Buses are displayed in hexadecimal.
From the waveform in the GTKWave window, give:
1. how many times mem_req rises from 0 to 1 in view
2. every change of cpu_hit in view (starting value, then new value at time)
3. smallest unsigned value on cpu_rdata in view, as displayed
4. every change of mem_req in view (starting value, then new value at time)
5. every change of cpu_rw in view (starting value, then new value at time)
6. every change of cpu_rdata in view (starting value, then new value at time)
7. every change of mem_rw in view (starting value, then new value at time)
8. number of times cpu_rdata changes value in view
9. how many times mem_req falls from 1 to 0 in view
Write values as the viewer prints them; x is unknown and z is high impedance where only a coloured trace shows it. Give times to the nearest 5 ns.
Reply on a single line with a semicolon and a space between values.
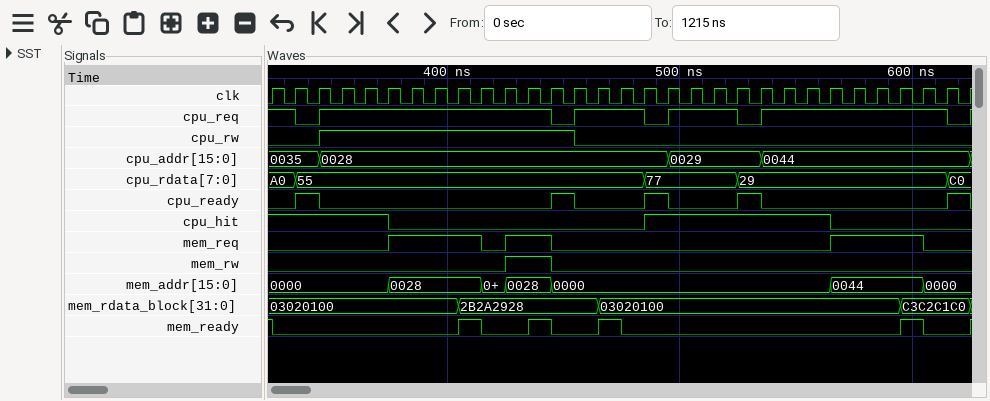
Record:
3; 1, 0 at 375 ns, 1 at 485 ns, 0 at 565 ns; 29; 0, 1 at 375 ns, 0 at 415 ns, 1 at 425 ns, 0 at 445 ns, 1 at 565 ns, 0 at 605 ns; 0, 1 at 345 ns, 0 at 455 ns; A0, 55 at 335 ns, 77 at 485 ns, 29 at 525 ns, C0 at 615 ns; 0, 1 at 425 ns, 0 at 445 ns; 4; 3
